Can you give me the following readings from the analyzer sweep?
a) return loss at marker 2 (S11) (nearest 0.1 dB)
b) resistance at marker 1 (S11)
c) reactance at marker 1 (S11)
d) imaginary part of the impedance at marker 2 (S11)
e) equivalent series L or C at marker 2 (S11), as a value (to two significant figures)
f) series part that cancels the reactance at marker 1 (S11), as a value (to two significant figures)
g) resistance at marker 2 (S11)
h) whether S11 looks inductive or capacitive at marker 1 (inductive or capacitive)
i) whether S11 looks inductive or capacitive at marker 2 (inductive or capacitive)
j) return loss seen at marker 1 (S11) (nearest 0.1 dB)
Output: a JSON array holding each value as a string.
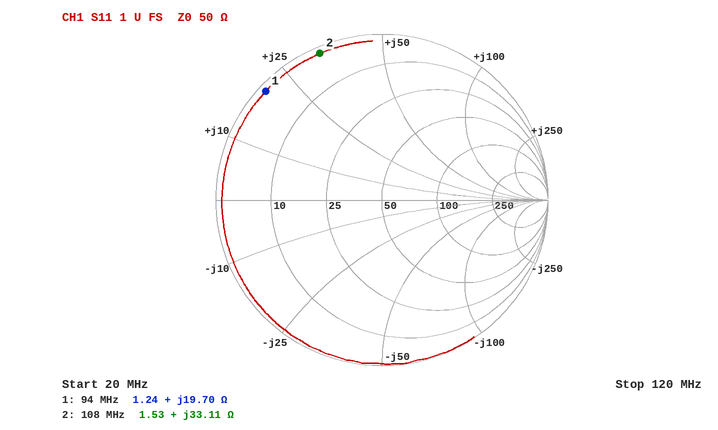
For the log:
["0.4 dB", "1.24 Ω", "+19.70 Ω", "+33.11 Ω", "49 nH", "86 pF", "1.53 Ω", "inductive", "inductive", "0.4 dB"]
